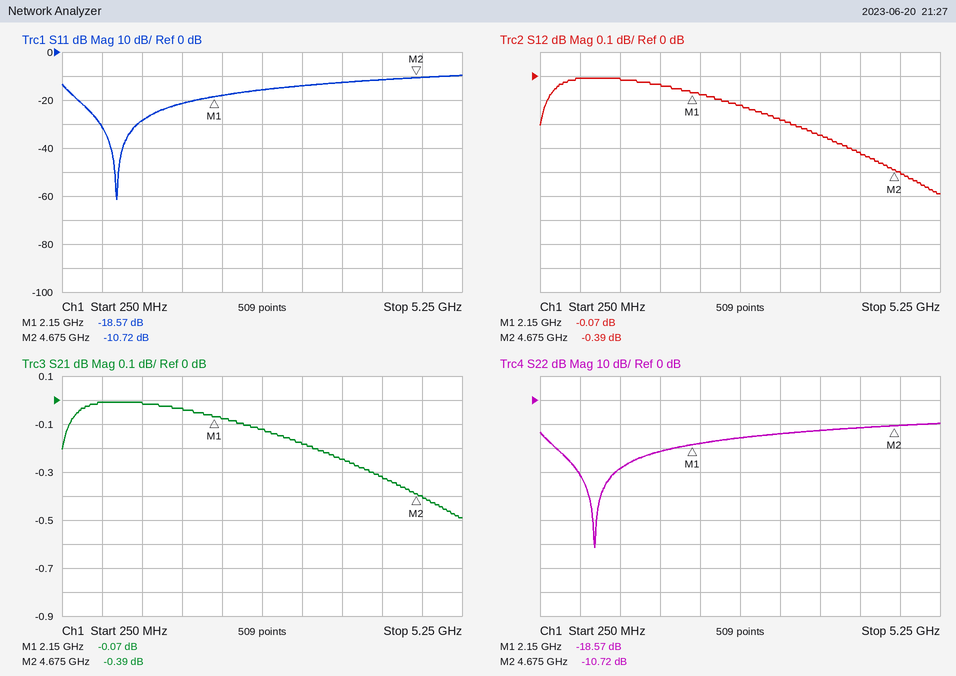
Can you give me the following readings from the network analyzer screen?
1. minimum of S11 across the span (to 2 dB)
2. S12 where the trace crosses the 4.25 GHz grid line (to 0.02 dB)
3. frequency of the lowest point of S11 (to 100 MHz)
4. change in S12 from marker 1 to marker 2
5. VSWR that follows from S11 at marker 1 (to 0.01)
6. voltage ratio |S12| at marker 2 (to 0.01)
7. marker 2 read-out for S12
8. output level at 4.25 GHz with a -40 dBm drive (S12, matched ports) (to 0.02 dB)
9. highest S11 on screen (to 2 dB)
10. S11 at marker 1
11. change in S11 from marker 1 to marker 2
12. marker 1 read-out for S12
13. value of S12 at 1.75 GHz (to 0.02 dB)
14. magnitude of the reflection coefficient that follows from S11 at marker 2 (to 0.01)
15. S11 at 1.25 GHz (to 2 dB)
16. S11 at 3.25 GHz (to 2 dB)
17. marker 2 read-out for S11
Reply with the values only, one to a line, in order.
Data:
-62 dB
-0.32 dB
900 MHz
-0.32 dB
1.27
0.96
-0.39 dB
-40.32 dBm
-10 dB
-18.57 dB
7.85 dB
-0.07 dB
-0.04 dB
0.29
-28 dB
-14 dB
-10.72 dB
